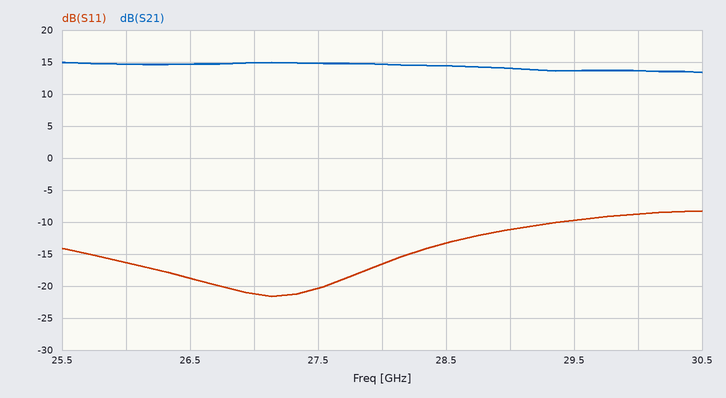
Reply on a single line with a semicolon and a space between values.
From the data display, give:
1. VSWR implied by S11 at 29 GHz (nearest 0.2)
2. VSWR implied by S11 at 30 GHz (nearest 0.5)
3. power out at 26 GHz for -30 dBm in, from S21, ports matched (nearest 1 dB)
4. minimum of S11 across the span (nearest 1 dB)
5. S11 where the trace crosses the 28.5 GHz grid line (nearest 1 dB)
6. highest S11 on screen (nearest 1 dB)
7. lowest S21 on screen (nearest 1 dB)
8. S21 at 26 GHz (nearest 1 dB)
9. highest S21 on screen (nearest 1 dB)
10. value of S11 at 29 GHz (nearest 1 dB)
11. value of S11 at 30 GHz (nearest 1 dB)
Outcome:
1.8; 2.0; -15 dBm; -22 dB; -13 dB; -8 dB; 13 dB; 15 dB; 15 dB; -11 dB; -9 dB
